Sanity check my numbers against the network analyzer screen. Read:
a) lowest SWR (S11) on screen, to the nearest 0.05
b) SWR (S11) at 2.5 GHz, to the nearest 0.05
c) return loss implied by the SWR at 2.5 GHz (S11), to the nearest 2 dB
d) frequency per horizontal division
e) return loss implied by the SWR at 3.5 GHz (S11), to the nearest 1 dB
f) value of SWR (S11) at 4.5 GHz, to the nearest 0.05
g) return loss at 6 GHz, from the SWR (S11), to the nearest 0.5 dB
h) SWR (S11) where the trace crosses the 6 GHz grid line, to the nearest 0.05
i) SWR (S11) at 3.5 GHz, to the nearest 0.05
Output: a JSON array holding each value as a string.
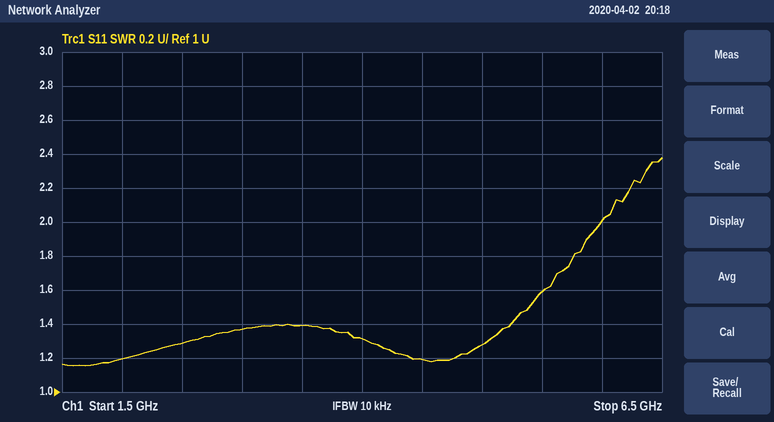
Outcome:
["1.15", "1.30", "18 dB", "500 MHz", "16 dB", "1.20", "9.5 dB", "2.00", "1.40"]
